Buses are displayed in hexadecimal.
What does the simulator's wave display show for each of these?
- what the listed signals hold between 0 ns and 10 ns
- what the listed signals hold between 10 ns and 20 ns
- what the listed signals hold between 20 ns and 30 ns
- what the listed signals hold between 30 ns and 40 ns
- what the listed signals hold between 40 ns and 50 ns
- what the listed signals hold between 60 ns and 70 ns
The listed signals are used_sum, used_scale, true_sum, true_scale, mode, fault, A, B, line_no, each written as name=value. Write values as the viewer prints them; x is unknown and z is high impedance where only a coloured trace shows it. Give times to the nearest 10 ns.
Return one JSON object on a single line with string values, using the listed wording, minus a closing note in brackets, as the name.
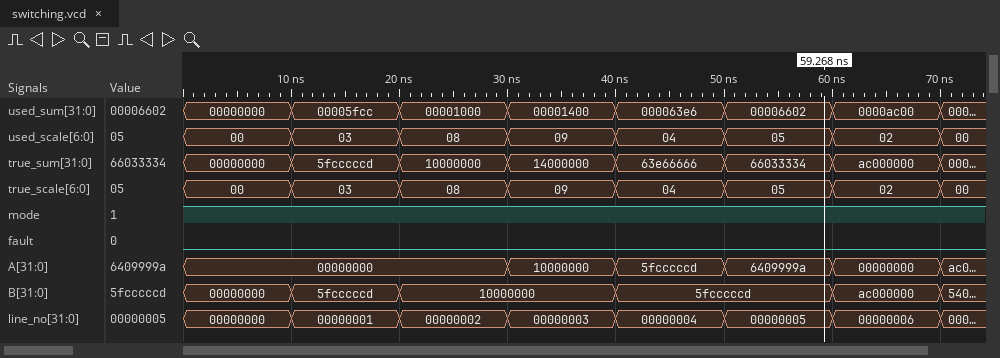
{"what the listed signals hold between 0 ns and 10 ns": "used_sum=00000000, used_scale=00, true_sum=00000000, true_scale=00, mode=1, fault=0, A=00000000, B=00000000, line_no=00000000", "what the listed signals hold between 10 ns and 20 ns": "used_sum=00005fcc, used_scale=03, true_sum=5fcccccd, true_scale=03, mode=1, fault=0, A=00000000, B=5fcccccd, line_no=00000001", "what the listed signals hold between 20 ns and 30 ns": "used_sum=00001000, used_scale=08, true_sum=10000000, true_scale=08, mode=1, fault=0, A=00000000, B=10000000, line_no=00000002", "what the listed signals hold between 30 ns and 40 ns": "used_sum=00001400, used_scale=09, true_sum=14000000, true_scale=09, mode=1, fault=0, A=10000000, B=10000000, line_no=00000003", "what the listed signals hold between 40 ns and 50 ns": "used_sum=000063e6, used_scale=04, true_sum=63e66666, true_scale=04, mode=1, fault=0, A=5fcccccd, B=5fcccccd, line_no=00000004", "what the listed signals hold between 60 ns and 70 ns": "used_sum=0000ac00, used_scale=02, true_sum=ac000000, true_scale=02, mode=1, fault=0, A=00000000, B=ac000000, line_no=00000006"}
